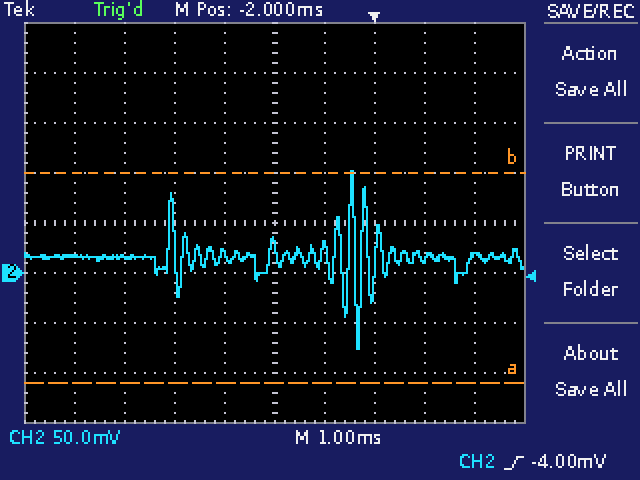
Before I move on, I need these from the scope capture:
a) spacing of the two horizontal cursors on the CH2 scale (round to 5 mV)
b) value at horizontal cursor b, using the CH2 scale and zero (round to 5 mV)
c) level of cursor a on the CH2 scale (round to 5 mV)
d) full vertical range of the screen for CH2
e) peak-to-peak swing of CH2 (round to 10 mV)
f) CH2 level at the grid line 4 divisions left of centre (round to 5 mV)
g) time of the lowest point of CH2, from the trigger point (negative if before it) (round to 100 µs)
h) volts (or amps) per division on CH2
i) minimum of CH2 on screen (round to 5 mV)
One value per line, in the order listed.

210 mV
100 mV
-110 mV
400 mV
180 mV
15 mV
-300 µs
50 mV
-75 mV
